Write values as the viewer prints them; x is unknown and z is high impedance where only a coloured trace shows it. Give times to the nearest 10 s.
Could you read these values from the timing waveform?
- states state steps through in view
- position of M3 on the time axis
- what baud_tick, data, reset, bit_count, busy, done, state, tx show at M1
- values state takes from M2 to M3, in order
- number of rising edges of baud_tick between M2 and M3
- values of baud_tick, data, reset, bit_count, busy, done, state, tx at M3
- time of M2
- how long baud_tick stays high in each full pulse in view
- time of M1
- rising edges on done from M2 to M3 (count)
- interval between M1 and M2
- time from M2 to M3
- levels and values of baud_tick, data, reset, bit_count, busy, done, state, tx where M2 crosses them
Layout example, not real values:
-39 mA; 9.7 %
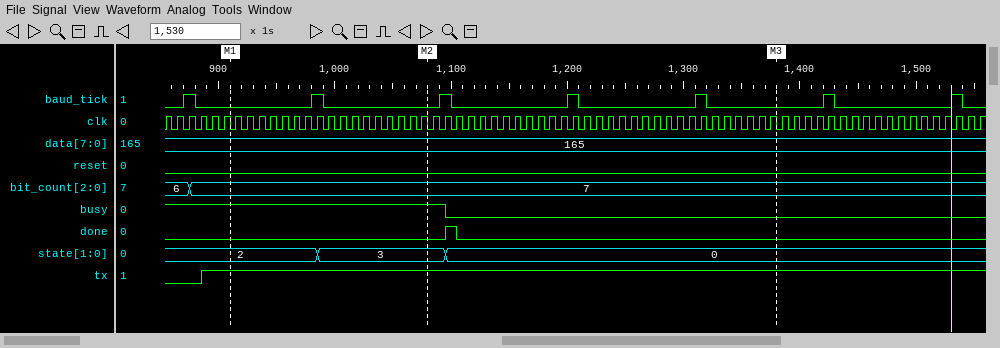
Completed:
2, 3, 0; 1380 s; baud_tick=0, data=165, reset=0, bit_count=7, busy=1, done=0, state=2, tx=1; 3, 0; 3; baud_tick=0, data=165, reset=0, bit_count=7, busy=0, done=0, state=0, tx=1; 1080 s; 10 s, 10 s, 10 s, 10 s, 10 s, 10 s, 10 s; 910 s; 1; 170 s; 300 s; baud_tick=0, data=165, reset=0, bit_count=7, busy=1, done=0, state=3, tx=1
